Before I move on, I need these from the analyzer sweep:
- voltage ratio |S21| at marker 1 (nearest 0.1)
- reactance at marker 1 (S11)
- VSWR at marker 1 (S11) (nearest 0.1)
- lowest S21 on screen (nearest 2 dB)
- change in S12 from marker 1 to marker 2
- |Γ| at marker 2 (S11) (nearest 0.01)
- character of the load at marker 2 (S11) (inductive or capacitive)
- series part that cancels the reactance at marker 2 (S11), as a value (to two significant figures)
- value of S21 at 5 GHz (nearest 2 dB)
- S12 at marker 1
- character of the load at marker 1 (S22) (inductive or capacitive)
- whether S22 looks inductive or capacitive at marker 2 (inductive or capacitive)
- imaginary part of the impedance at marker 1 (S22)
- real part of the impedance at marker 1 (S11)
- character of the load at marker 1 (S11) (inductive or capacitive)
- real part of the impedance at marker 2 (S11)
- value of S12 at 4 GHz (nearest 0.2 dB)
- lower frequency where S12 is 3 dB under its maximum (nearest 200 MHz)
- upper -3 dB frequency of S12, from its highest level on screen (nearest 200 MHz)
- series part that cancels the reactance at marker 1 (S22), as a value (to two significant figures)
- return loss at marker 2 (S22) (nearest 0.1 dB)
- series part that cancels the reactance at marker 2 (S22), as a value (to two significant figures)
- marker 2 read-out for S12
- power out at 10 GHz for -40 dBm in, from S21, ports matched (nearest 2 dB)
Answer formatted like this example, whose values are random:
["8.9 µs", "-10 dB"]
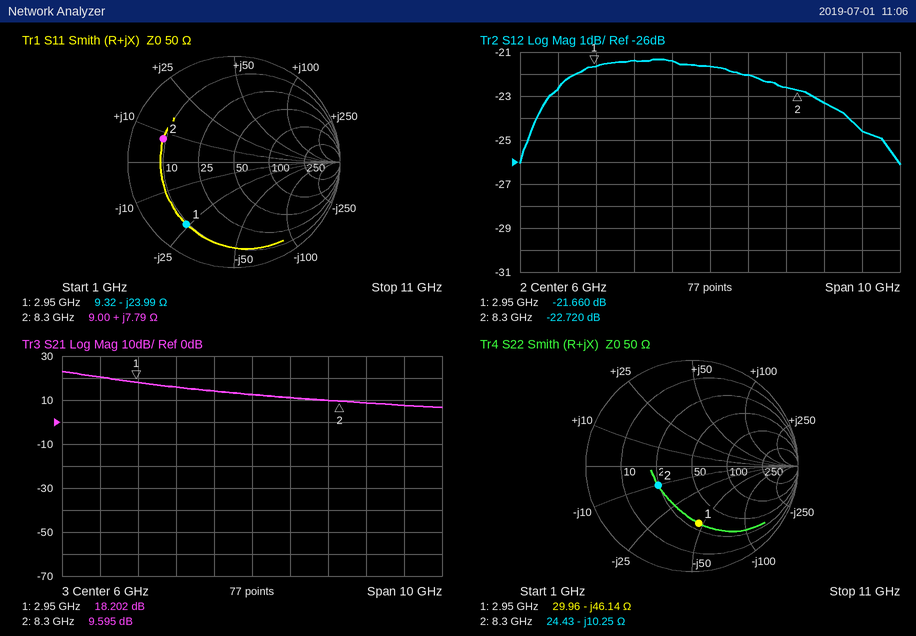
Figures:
["8.1", "-23.99 Ω", "6.6", "6 dB", "-1.060 dB", "0.70", "inductive", "2.5 pF", "14 dB", "-21.660 dB", "capacitive", "capacitive", "-46.14 Ω", "9.32 Ω", "capacitive", "9.00 Ω", "-21.4 dB", "1.4 GHz", "9.8 GHz", "2.5 nH", "8.7 dB", "200 pH", "-22.720 dB", "-32 dBm"]
